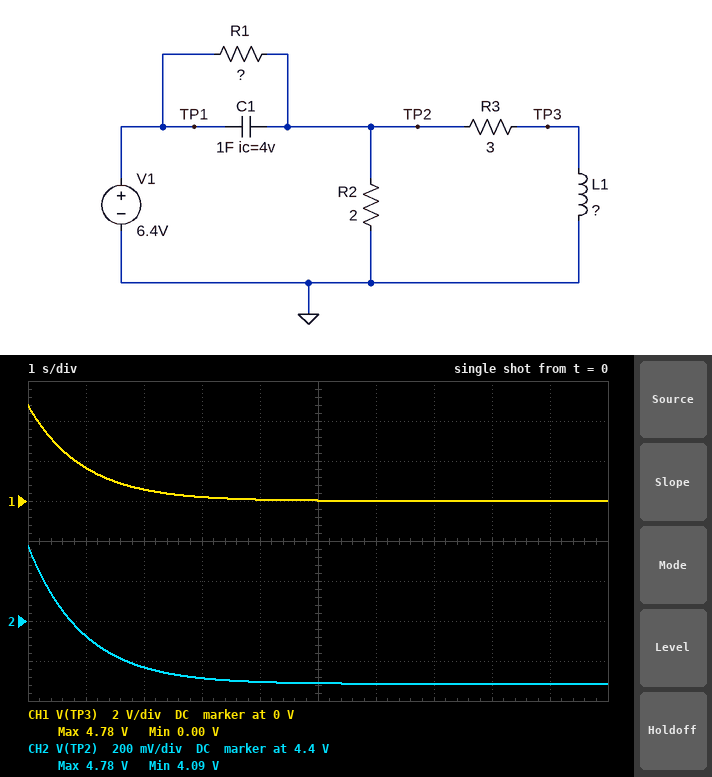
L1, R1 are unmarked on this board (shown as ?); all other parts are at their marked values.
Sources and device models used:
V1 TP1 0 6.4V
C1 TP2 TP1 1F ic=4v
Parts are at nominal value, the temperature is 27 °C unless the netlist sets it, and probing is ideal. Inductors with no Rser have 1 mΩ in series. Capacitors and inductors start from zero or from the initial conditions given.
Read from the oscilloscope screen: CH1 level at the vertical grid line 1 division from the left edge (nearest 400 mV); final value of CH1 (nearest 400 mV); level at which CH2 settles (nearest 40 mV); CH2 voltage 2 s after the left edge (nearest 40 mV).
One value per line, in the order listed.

1.6 V
0 V
4.08 V
4.16 V
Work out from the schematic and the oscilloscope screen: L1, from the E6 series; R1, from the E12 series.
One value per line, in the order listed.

3.3 H
0.68 Ω
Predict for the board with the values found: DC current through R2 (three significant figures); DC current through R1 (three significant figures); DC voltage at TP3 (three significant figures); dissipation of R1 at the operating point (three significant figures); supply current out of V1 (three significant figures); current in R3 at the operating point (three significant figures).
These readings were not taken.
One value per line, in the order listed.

2.04 A
3.40 A
1.36 mV
7.88 W
3.40 A
1.36 A
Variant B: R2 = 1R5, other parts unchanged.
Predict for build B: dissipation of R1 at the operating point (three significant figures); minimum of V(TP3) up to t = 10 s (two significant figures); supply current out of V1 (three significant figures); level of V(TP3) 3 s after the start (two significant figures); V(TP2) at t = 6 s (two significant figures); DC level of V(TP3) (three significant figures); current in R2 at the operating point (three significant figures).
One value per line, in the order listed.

9.87 W
1.4 mV
3.81 A
190 mV
3.8 V
1.27 mV
2.54 A
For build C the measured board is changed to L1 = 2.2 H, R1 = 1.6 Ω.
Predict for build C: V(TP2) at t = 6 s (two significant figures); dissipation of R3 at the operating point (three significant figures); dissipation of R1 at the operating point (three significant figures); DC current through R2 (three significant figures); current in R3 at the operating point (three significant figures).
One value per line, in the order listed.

2.7 V
2.51 W
8.36 W
1.37 A
914 mA
